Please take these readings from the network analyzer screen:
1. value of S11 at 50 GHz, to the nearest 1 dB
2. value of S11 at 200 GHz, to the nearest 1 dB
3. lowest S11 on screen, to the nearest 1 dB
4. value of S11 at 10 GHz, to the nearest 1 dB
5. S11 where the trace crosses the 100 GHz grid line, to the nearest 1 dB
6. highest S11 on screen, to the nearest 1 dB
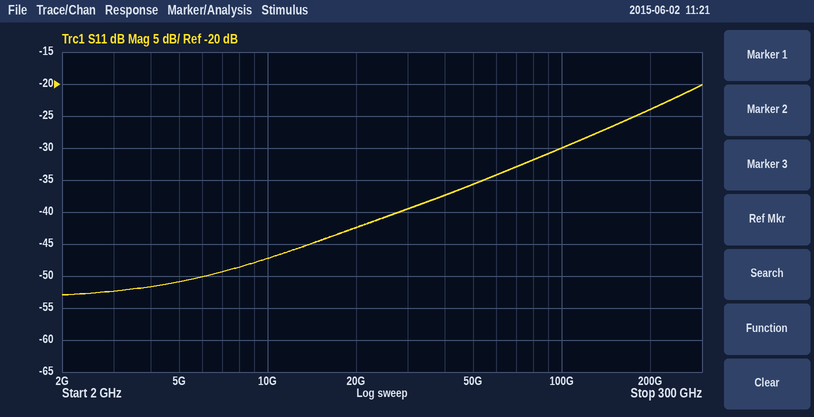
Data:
-36 dB
-24 dB
-53 dB
-47 dB
-30 dB
-20 dB
